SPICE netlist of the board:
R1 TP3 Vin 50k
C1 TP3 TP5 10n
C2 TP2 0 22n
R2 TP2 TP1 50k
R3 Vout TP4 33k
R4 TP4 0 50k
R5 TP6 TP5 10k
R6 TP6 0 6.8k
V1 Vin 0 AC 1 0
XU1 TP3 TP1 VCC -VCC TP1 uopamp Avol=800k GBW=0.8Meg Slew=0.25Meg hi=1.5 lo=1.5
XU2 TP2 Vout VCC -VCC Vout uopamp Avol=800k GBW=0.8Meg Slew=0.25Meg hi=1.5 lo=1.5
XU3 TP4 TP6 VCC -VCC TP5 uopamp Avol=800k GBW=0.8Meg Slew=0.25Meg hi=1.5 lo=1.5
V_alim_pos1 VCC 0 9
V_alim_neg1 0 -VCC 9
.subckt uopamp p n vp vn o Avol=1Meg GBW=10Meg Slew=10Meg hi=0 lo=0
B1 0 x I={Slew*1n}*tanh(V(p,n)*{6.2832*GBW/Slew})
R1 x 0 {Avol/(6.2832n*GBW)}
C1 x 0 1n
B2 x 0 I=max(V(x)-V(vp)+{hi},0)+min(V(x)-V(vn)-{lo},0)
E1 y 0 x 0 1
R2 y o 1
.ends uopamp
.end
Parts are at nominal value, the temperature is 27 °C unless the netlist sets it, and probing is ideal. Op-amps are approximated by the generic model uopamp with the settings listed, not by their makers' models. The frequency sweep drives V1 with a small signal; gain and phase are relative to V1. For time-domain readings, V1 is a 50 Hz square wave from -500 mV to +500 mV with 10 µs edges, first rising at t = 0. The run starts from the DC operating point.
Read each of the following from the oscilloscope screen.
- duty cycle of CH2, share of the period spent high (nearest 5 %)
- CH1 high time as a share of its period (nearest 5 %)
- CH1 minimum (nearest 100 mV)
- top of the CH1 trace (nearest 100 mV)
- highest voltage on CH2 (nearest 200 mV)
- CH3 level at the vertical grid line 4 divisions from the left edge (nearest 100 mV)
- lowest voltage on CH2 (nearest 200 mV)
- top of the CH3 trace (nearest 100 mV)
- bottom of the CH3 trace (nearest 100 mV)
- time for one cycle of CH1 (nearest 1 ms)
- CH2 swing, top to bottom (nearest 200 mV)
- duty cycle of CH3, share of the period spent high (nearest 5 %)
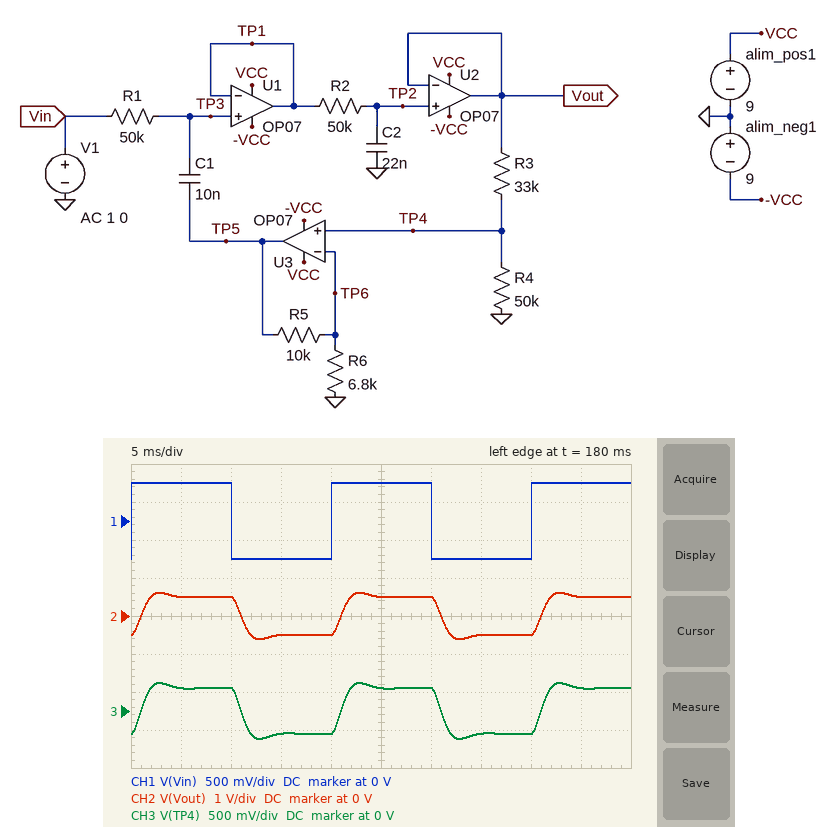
50 %
50 %
-500 mV
500 mV
600 mV
-300 mV
-600 mV
400 mV
-400 mV
20 ms
1.2 V
50 %
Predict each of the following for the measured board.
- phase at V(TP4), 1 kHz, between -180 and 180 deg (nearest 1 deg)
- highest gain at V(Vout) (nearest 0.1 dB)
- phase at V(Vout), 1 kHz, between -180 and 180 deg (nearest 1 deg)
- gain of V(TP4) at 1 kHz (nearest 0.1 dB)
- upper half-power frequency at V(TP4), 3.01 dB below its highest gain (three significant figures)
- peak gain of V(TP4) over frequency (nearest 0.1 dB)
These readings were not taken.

-166 deg
0.5 dB
-166 deg
-31.0 dB
242 Hz
-3.9 dB
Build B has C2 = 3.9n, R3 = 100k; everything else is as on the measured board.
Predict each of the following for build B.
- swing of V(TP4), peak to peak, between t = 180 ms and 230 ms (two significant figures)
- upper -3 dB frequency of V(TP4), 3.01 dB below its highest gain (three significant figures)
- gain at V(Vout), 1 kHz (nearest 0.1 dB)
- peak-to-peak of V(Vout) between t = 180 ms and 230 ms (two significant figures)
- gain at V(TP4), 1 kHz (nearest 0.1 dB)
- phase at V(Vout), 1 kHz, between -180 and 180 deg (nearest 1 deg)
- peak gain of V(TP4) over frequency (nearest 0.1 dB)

470 mV
601 Hz
-10.6 dB
1.4 V
-20.1 dB
-148 deg
-7.7 dB
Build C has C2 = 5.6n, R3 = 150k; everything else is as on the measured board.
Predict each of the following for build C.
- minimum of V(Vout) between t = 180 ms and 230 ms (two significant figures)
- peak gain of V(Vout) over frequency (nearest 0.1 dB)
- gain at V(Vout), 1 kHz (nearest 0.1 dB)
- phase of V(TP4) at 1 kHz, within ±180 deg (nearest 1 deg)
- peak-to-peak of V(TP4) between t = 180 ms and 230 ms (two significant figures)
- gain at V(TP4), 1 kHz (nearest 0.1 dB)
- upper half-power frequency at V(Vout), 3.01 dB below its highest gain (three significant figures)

-580 mV
0.2 dB
-14.7 dB
-147 deg
290 mV
-26.7 dB
463 Hz
